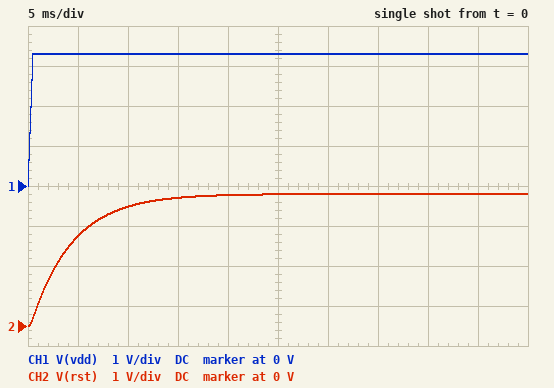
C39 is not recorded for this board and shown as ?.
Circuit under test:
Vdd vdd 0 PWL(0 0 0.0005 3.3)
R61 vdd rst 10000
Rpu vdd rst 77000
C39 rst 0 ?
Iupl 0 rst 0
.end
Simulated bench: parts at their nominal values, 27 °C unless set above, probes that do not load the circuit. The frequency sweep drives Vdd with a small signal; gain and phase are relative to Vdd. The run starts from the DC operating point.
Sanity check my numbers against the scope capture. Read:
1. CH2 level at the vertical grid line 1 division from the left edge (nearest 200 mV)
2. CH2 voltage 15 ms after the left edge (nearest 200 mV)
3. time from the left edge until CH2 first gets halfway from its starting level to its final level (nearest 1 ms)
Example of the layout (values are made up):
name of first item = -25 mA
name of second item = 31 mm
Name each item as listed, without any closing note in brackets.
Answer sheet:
CH2 level at the vertical grid line 1 division from the left edge = 2.2 V
CH2 voltage 15 ms after the left edge = 3.2 V
time from the left edge until CH2 first gets halfway from its starting level to its final level = 3 ms
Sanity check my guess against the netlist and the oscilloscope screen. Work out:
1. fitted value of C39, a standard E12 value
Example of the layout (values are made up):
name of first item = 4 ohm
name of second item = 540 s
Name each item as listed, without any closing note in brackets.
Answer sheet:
fitted value of C39, a standard E12 value = 470 nF
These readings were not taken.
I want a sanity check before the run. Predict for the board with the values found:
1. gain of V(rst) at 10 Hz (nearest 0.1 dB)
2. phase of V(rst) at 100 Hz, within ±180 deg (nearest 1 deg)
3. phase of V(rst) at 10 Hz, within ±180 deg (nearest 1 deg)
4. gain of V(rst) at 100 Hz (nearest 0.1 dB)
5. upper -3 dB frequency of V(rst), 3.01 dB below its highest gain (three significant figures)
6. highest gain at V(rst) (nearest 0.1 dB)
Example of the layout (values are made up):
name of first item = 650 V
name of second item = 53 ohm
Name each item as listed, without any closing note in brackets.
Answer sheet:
gain of V(rst) at 10 Hz = -0.3 dB
phase of V(rst) at 100 Hz, within ±180 deg = -69 deg
phase of V(rst) at 10 Hz, within ±180 deg = -15 deg
gain of V(rst) at 100 Hz = -8.9 dB
upper -3 dB frequency of V(rst), 3.01 dB below its highest gain = 38.3 Hz
highest gain at V(rst) = 0 dB
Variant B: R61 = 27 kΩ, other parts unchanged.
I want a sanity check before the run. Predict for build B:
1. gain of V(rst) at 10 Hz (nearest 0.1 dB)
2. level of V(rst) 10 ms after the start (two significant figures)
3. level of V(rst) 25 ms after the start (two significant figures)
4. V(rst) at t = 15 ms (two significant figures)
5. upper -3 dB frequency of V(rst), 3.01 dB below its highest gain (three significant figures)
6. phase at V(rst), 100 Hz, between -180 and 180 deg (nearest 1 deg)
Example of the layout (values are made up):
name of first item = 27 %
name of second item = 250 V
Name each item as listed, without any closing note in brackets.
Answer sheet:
gain of V(rst) at 10 Hz = -1.3 dB
level of V(rst) 10 ms after the start = 2.1 V
level of V(rst) 25 ms after the start = 3.1 V
V(rst) at t = 15 ms = 2.6 V
upper -3 dB frequency of V(rst), 3.01 dB below its highest gain = 16.9 Hz
phase at V(rst), 100 Hz, between -180 and 180 deg = -80 deg
